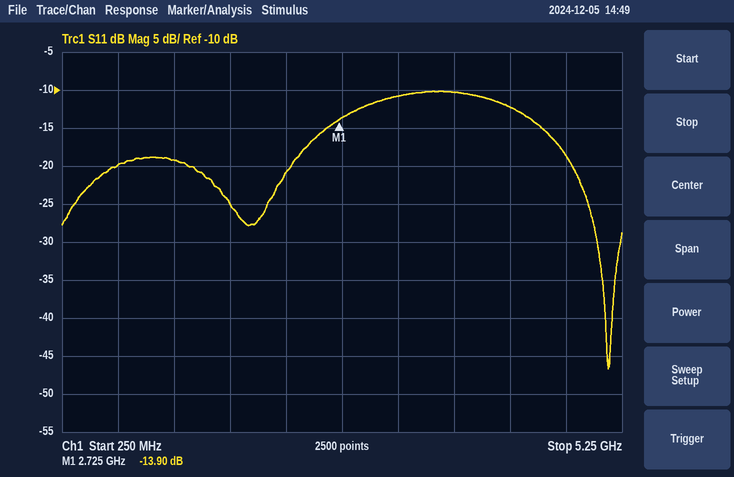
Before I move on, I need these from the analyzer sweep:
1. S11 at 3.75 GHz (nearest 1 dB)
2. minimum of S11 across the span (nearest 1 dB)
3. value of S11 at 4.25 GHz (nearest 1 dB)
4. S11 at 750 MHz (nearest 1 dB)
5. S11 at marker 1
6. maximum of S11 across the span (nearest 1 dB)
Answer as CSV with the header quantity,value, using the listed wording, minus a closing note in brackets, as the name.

quantity,value
S11 at 3.75 GHz,-10 dB
minimum of S11 across the span,-47 dB
value of S11 at 4.25 GHz,-12 dB
S11 at 750 MHz,-20 dB
S11 at marker 1,-13.90 dB
maximum of S11 across the span,-10 dB
